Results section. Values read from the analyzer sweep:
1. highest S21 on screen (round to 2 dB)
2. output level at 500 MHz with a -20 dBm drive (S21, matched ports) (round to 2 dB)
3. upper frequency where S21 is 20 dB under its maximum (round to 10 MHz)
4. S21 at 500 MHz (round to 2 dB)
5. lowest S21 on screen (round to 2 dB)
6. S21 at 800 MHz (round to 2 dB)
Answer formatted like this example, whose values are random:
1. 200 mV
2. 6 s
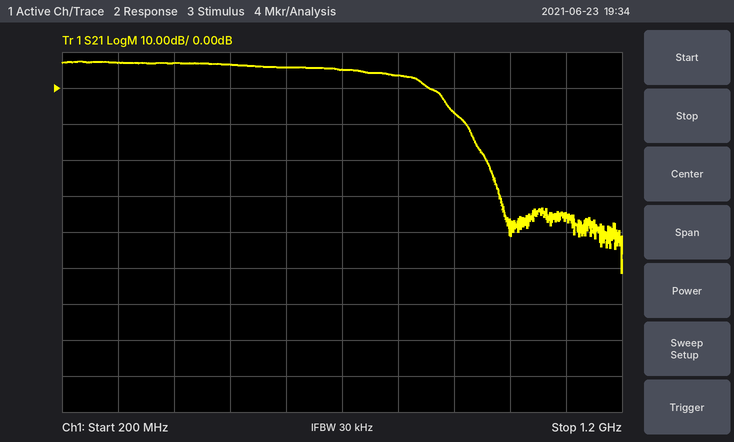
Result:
1. 8 dB
2. -14 dBm
3. 930 MHz
4. 6 dB
5. -52 dB
6. 4 dB
